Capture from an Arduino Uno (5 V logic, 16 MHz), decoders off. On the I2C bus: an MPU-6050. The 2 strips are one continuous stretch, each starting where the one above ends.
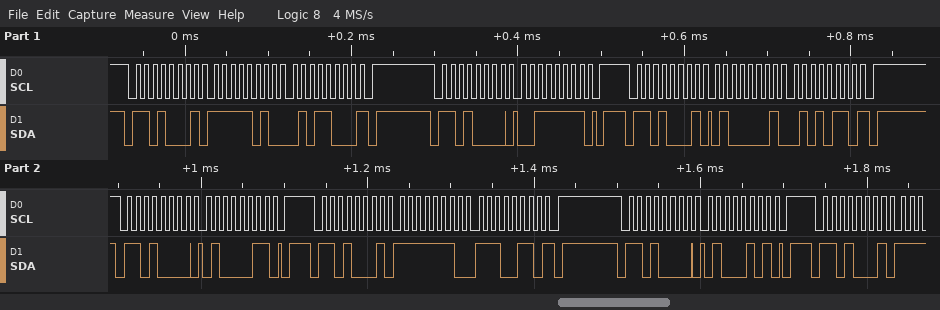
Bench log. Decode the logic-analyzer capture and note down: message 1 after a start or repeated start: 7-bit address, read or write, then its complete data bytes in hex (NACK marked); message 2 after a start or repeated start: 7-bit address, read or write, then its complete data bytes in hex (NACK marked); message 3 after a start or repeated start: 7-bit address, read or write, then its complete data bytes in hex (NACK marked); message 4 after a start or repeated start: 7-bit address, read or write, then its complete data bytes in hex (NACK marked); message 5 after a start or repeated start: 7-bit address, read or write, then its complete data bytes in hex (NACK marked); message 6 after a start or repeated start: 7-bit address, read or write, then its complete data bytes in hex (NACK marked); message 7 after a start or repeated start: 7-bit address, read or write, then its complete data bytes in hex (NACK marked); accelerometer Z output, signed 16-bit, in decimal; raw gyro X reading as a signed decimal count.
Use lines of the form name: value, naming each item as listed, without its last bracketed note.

message 1 after a start or repeated start: 7-bit address, read or write, then its complete data bytes in hex: 0x68 read: FA 58 NACK
message 2 after a start or repeated start: 7-bit address, read or write, then its complete data bytes in hex: 0x68 write: 3F
message 3 after a start or repeated start: 7-bit address, read or write, then its complete data bytes in hex: 0x68 read: 41 56 NACK
message 4 after a start or repeated start: 7-bit address, read or write, then its complete data bytes in hex: 0x68 write: 43
message 5 after a start or repeated start: 7-bit address, read or write, then its complete data bytes in hex: 0x68 read: FE E6 NACK
message 6 after a start or repeated start: 7-bit address, read or write, then its complete data bytes in hex: 0x68 write: 45
message 7 after a start or repeated start: 7-bit address, read or write, then its complete data bytes in hex: 0x68 read
accelerometer Z output, signed 16-bit, in decimal: 16726
raw gyro X reading as a signed decimal count: -282
